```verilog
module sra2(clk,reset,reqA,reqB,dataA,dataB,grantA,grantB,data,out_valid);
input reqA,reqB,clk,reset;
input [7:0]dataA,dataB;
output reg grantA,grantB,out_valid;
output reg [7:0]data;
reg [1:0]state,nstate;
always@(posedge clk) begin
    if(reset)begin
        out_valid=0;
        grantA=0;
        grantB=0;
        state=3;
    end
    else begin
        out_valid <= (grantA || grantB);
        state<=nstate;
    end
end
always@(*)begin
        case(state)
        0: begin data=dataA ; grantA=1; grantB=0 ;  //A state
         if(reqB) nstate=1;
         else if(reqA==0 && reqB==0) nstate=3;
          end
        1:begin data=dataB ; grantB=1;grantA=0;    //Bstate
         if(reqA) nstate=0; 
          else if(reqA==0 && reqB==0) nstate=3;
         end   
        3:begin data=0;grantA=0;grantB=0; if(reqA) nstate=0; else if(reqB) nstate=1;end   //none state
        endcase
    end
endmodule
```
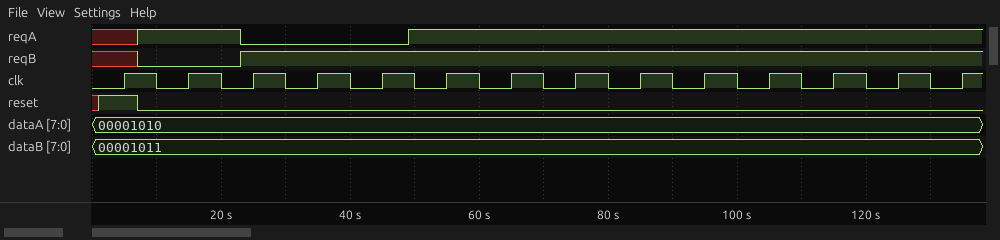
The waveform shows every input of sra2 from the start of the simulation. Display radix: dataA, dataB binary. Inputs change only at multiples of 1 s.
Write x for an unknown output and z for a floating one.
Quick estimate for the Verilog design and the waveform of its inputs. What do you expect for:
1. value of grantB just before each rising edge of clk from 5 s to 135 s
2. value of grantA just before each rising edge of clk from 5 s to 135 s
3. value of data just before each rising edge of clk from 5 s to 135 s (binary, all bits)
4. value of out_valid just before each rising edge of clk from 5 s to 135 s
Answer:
x 0 0 1 1 1 0 1 0 1 0 1 0 1
x 0 1 0 0 0 1 0 1 0 1 0 1 0
x, 00000000, 00001010, 00001011, 00001011, 00001011, 00001010, 00001011, 00001010, 00001011, 00001010, 00001011, 00001010, 00001011
x 0 0 1 1 1 1 1 1 1 1 1 1 1
